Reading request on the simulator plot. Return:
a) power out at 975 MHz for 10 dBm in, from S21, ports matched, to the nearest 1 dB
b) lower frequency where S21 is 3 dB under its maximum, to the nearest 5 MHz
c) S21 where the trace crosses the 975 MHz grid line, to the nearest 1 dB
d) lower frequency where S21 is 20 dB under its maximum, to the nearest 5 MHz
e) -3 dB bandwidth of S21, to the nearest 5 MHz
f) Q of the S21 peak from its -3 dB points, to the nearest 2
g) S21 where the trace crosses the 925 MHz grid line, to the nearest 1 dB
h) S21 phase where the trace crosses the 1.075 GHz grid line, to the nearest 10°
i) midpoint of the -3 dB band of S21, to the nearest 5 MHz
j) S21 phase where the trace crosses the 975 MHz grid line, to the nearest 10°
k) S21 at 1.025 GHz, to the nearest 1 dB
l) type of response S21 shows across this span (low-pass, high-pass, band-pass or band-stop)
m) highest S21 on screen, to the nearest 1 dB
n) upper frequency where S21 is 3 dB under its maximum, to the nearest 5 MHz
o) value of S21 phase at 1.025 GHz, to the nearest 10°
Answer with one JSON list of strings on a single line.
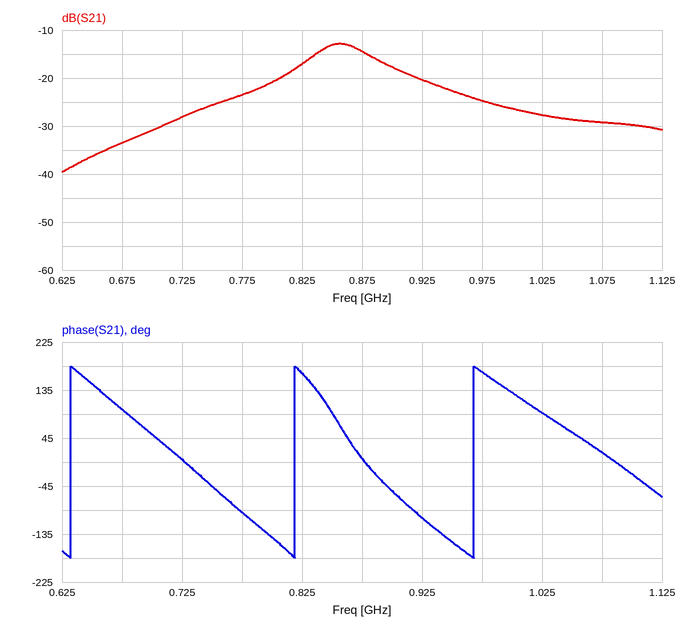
["-15 dBm", "830 MHz", "-25 dB", "680 MHz", "55 MHz", "16", "-20 dB", "20°", "860 MHz", "170°", "-28 dB", "band-pass", "-13 dB", "885 MHz", "90°"]
